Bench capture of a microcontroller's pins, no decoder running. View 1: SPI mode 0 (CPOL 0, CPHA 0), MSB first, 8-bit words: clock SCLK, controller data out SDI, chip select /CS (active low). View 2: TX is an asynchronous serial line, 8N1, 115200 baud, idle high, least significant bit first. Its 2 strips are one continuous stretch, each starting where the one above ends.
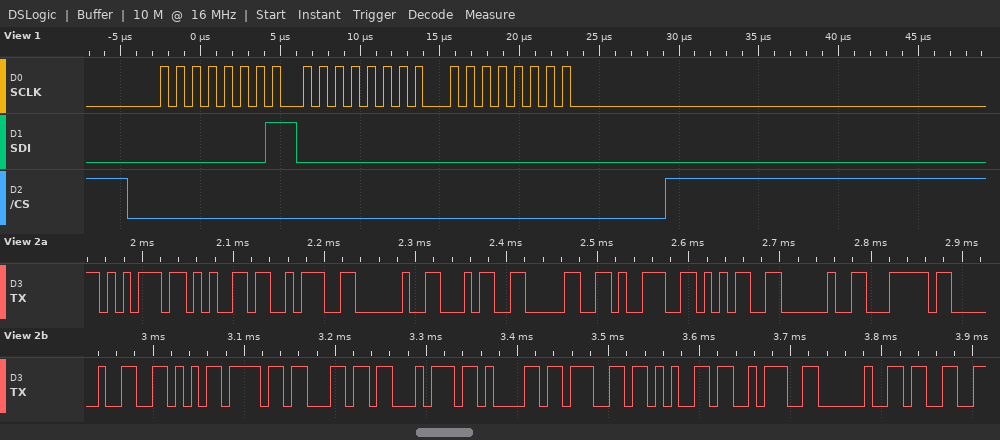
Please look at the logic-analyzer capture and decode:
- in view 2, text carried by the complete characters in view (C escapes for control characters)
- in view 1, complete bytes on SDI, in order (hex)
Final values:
"ue: 4095 | Voltage: 3"
01 00 00
